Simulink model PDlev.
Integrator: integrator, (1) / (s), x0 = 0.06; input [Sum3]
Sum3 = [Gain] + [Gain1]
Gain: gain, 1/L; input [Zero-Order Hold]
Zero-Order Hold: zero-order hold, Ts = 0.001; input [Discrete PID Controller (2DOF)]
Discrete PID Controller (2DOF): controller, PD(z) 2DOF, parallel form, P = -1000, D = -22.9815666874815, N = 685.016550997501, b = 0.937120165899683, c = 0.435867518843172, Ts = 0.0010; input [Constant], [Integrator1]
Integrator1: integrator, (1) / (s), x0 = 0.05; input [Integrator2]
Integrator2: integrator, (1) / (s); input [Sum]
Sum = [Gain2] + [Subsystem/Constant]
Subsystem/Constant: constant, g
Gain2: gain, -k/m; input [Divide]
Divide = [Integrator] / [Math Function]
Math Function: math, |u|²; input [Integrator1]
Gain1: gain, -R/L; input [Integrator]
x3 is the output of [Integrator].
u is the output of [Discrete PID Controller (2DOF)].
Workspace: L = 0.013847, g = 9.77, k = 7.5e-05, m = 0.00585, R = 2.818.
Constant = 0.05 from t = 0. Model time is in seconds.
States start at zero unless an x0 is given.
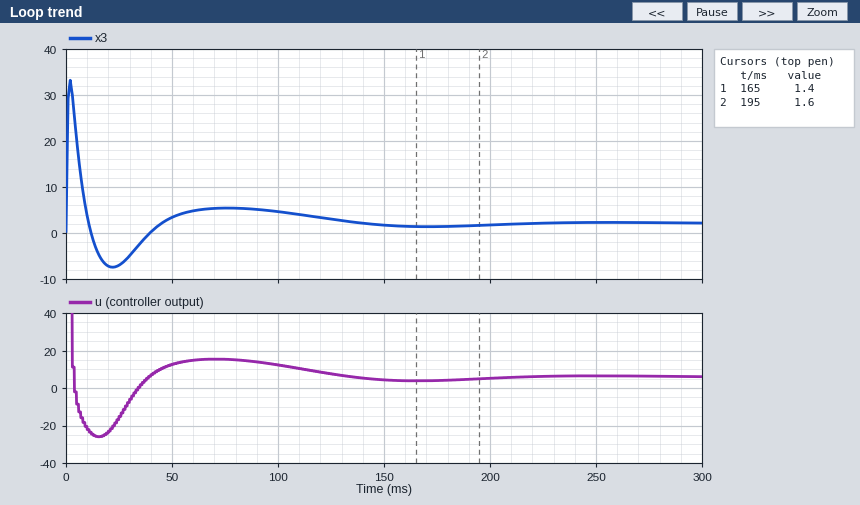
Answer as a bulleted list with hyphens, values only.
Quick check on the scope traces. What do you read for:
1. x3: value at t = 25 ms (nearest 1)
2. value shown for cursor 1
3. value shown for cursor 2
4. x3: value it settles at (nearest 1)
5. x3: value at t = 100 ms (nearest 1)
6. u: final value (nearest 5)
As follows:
- -7
- 1.4
- 1.6
- 2
- 5
- 5
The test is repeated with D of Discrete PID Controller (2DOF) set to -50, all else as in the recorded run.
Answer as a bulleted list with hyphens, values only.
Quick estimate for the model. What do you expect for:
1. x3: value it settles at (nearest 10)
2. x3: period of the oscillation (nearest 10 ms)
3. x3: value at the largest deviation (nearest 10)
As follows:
- 0
- 30 ms
- 70
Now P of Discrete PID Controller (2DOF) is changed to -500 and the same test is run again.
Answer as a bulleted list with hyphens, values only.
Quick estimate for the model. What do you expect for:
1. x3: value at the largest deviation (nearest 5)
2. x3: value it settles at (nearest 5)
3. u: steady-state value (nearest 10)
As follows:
- 35
- 5
- 10
